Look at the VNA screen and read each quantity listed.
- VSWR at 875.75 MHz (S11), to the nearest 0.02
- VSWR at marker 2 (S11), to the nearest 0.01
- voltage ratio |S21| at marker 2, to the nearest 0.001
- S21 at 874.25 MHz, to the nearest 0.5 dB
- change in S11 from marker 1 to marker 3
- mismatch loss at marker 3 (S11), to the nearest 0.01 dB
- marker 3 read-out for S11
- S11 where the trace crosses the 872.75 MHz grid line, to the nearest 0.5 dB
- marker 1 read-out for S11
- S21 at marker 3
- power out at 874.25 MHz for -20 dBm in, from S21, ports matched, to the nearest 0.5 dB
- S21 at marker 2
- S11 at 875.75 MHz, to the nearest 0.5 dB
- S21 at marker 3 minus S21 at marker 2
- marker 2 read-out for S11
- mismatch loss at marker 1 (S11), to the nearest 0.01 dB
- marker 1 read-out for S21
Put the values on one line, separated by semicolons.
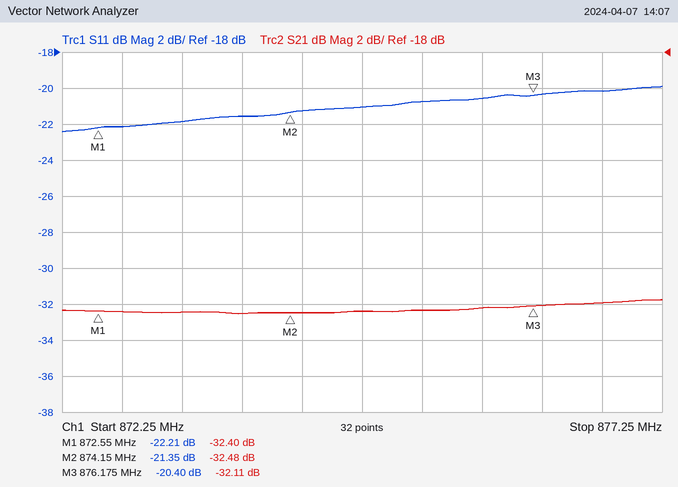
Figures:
1.20; 1.19; 0.024; -32.5 dB; 1.81 dB; 0.04 dB; -20.40 dB; -22.0 dB; -22.21 dB; -32.11 dB; -52.5 dBm; -32.48 dB; -20.5 dB; 0.37 dB; -21.35 dB; 0.03 dB; -32.40 dB
